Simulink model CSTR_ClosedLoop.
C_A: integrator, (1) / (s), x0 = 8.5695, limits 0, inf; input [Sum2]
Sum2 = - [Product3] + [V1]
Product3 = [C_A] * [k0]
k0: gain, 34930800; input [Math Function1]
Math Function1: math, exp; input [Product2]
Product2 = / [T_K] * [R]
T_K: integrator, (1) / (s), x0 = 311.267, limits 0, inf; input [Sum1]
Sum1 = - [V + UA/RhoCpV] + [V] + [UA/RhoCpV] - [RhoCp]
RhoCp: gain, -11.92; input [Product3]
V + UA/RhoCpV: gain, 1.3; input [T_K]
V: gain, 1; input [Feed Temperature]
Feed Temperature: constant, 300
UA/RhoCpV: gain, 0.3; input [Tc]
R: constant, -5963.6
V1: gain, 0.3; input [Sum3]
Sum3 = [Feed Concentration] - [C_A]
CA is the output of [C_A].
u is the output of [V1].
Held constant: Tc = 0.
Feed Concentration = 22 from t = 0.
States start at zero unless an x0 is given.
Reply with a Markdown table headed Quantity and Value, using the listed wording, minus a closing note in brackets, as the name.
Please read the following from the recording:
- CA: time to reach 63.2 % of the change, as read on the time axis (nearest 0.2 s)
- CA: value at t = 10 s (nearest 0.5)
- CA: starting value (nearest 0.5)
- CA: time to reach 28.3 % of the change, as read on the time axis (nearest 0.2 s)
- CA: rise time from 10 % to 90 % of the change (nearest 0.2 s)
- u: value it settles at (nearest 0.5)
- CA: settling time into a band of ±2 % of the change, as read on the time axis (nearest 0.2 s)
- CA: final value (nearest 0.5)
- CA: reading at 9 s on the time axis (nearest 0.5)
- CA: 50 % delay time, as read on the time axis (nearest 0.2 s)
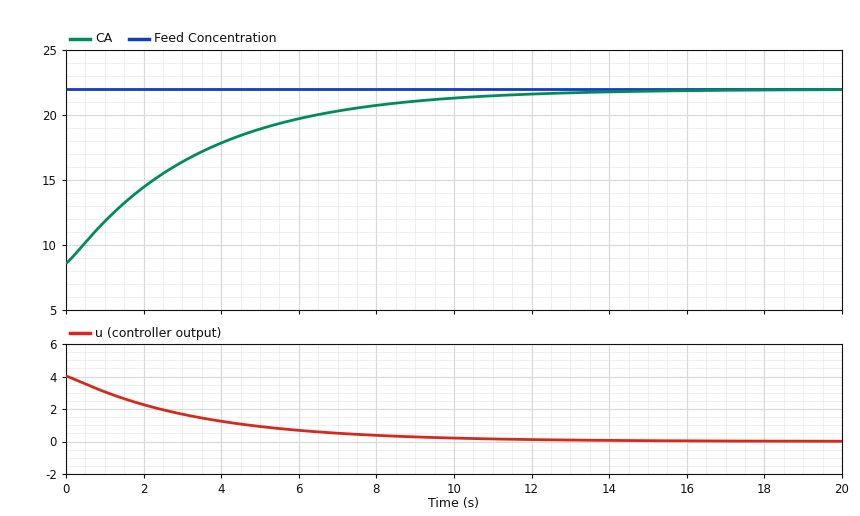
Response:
| Quantity | Value |
|---|---|
| CA: time to reach 63.2 % of the change, as read on the time axis | 3.4 s |
| CA: value at t = 10 s | 21.5 |
| CA: starting value | 8.5 |
| CA: time to reach 28.3 % of the change, as read on the time axis | 1.2 s |
| CA: rise time from 10 % to 90 % of the change | 7.4 s |
| u: value it settles at | 0.0 |
| CA: settling time into a band of ±2 % of the change, as read on the time axis | 13.2 s |
| CA: final value | 22.0 |
| CA: reading at 9 s on the time axis | 21.0 |
| CA: 50 % delay time, as read on the time axis | 2.4 s |
